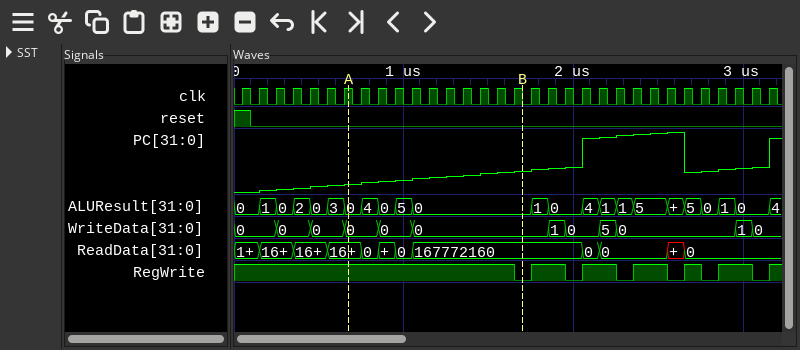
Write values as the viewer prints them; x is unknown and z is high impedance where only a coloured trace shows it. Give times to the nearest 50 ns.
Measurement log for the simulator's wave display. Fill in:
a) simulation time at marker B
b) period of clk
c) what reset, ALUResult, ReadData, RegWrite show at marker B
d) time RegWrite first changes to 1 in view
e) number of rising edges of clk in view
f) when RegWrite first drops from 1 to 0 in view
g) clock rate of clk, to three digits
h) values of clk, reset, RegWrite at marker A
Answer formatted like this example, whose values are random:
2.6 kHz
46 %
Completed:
1700 ns
100 ns
reset=0, ALUResult=0, ReadData=167772160, RegWrite=0
1750 ns
32
1650 ns
10.0 MHz
clk=1, reset=0, RegWrite=1
